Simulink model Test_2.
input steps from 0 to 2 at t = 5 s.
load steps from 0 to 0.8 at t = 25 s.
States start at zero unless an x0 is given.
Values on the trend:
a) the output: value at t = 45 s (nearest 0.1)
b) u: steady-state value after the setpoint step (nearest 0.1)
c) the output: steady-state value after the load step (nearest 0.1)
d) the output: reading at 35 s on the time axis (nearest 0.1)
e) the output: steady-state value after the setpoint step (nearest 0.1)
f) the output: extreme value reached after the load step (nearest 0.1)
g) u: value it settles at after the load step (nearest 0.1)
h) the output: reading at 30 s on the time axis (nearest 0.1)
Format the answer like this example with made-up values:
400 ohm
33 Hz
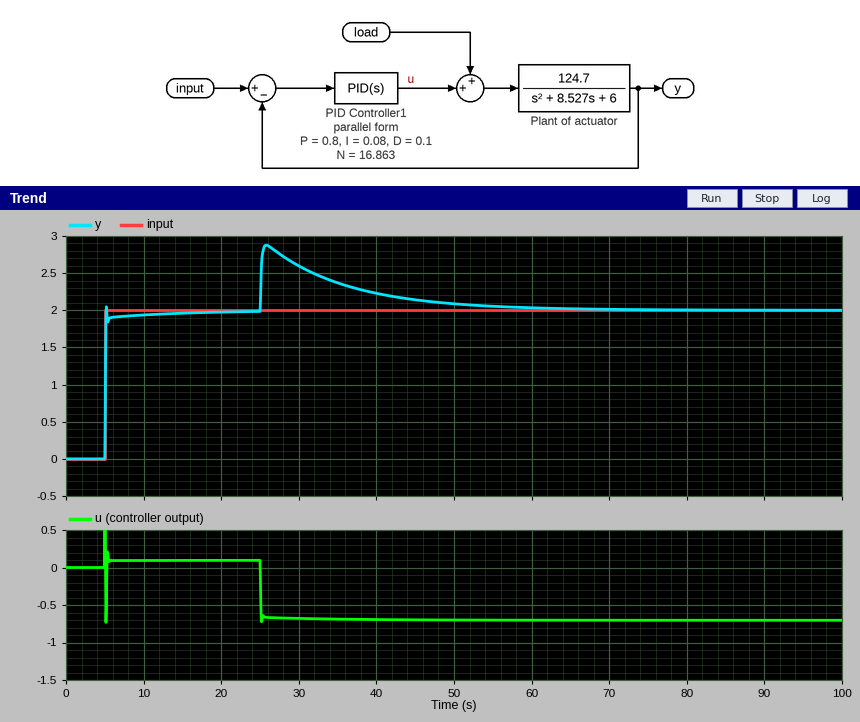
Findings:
2.1
0.1
2.0
2.4
2.0
2.9
-0.7
2.6
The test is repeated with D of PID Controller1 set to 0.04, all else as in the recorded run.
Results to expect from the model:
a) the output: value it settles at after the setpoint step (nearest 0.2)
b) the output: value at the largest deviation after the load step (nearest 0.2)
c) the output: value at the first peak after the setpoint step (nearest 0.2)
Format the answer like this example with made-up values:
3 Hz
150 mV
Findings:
2.0
3.0
2.2
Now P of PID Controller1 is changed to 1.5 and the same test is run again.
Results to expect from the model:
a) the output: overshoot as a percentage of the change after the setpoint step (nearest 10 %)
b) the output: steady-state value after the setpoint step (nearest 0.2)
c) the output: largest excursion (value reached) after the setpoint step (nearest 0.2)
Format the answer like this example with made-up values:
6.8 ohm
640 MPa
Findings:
20 %
2.0
2.4
